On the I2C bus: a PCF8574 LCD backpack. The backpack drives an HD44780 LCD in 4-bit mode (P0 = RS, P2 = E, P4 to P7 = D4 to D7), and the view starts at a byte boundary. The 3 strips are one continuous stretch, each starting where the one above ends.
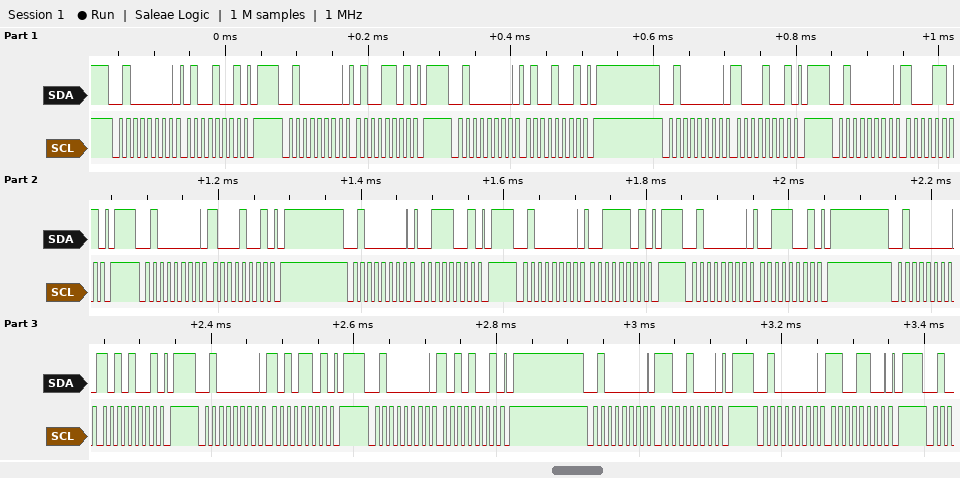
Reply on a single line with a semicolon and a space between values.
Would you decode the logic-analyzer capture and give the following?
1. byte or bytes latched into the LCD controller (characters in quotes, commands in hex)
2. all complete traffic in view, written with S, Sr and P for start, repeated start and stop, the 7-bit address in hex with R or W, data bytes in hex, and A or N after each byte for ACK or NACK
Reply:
'H' ':'; S 20W A 49 A P S 20W A 4D A P S 20W A 49 A P S 20W A 89 A P S 20W A 8D A P S 20W A 89 A P S 20W A 39 A P S 20W A 3D A P S 20W A 39 A P S 20W A A9 A P S 20W A AD A P S 20W A A9 A P S 20W A C8 A P S 20W A CC A P
